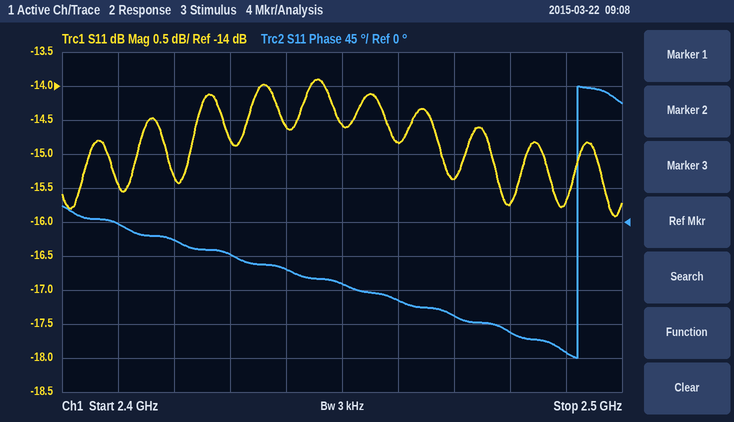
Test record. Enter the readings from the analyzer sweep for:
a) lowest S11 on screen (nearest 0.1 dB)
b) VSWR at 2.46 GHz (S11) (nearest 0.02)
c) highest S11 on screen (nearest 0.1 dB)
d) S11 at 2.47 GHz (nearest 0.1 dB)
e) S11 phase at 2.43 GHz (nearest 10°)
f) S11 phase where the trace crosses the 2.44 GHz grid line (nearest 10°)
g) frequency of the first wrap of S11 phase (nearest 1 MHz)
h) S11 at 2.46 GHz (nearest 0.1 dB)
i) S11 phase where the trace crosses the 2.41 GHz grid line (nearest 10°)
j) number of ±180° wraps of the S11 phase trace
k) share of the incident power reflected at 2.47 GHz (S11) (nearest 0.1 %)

-15.9 dB
1.44
-13.9 dB
-15.4 dB
-40°
-60°
2.492 GHz
-14.8 dB
0°
1
2.9 %
